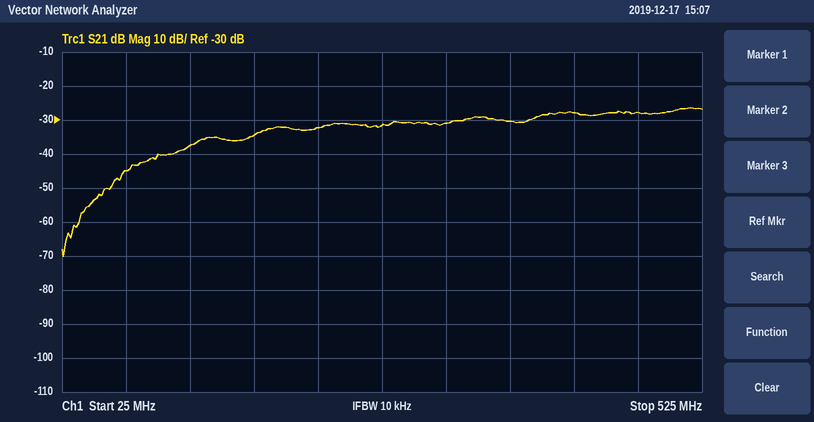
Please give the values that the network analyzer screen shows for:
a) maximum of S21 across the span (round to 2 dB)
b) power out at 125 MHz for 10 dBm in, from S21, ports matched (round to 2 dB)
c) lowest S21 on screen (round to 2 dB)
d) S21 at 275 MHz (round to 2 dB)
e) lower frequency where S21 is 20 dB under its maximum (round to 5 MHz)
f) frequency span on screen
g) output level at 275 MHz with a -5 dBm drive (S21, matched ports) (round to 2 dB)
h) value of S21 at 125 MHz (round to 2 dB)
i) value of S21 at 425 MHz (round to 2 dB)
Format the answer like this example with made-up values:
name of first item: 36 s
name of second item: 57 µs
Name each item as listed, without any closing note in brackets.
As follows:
maximum of S21 across the span: -26 dB
power out at 125 MHz for 10 dBm in, from S21, ports matched: -28 dBm
lowest S21 on screen: -70 dB
S21 at 275 MHz: -32 dB
lower frequency where S21 is 20 dB under its maximum: 70 MHz
frequency span on screen: 500 MHz
output level at 275 MHz with a -5 dBm drive (S21, matched ports): -36 dBm
value of S21 at 125 MHz: -38 dB
value of S21 at 425 MHz: -28 dB
